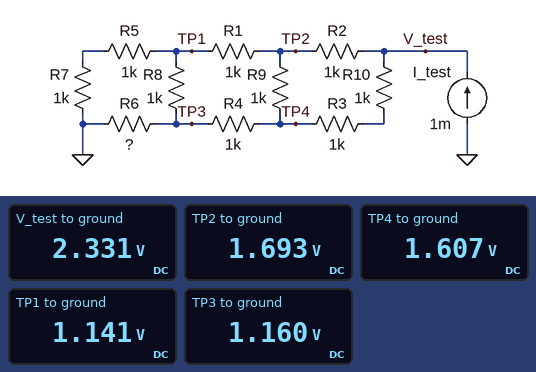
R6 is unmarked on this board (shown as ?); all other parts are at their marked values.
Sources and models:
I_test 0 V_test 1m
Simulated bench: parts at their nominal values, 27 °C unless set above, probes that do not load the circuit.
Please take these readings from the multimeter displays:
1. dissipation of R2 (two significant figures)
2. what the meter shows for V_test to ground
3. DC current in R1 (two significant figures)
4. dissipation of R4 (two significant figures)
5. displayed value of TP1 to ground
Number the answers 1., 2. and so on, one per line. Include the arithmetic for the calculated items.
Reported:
1. (2.331 V - 1.693 V)^2 / 1 kΩ = 410 µW
2. 2.331 V
3. (1.693 V - 1.141 V) / 1 kΩ = 550 µA
4. (1.607 V - 1.16 V)^2 / 1 kΩ = 200 µW
5. 1.141 V
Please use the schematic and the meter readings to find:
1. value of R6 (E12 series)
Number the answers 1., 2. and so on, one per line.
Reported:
1. 2.7 kΩ
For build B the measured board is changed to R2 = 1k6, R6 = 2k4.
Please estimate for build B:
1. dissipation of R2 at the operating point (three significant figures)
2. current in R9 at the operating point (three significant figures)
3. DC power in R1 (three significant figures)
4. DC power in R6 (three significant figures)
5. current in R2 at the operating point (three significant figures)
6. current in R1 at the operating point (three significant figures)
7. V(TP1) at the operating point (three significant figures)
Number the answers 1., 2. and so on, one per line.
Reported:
1. 481 µW
2. 26.0 µA
3. 273 µW
4. 505 µW
5. 548 µA
6. 522 µA
7. 1.08 V
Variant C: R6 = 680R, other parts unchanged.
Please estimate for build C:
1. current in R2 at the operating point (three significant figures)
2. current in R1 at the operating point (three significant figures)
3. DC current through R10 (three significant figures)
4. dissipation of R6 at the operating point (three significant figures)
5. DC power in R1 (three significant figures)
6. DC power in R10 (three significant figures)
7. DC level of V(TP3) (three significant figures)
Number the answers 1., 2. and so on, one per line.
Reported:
1. 621 µA
2. 484 µA
3. 379 µA
4. 318 µW
5. 235 µW
6. 144 µW
7. 465 mV
